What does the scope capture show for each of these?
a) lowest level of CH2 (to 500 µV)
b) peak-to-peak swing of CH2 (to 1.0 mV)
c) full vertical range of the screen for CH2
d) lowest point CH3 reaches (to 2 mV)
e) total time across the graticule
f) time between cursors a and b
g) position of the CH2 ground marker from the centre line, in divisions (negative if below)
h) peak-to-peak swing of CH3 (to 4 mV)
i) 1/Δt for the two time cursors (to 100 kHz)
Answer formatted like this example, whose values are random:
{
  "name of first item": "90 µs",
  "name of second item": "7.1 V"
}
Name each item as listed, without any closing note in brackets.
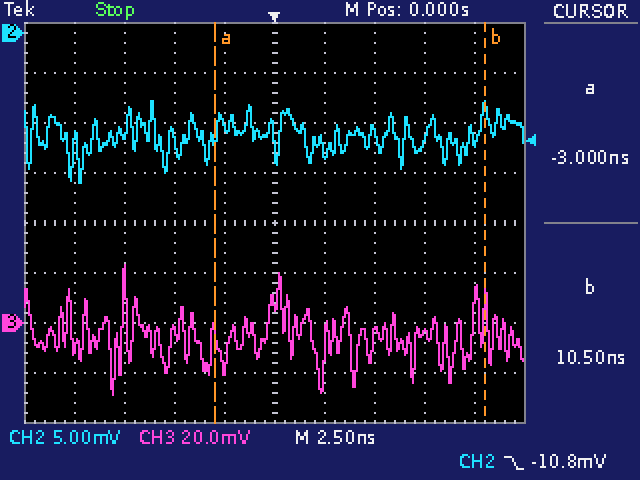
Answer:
{
  "lowest level of CH2": "-15.0 mV",
  "peak-to-peak swing of CH2": "8.0 mV",
  "full vertical range of the screen for CH2": "40 mV",
  "lowest point CH3 reaches": "-28 mV",
  "total time across the graticule": "25 ns",
  "time between cursors a and b": "13.50 ns",
  "position of the CH2 ground marker from the centre line, in divisions": "+3.8 div",
  "peak-to-peak swing of CH3": "52 mV",
  "1/Δt for the two time cursors": "74.1 MHz"
}
